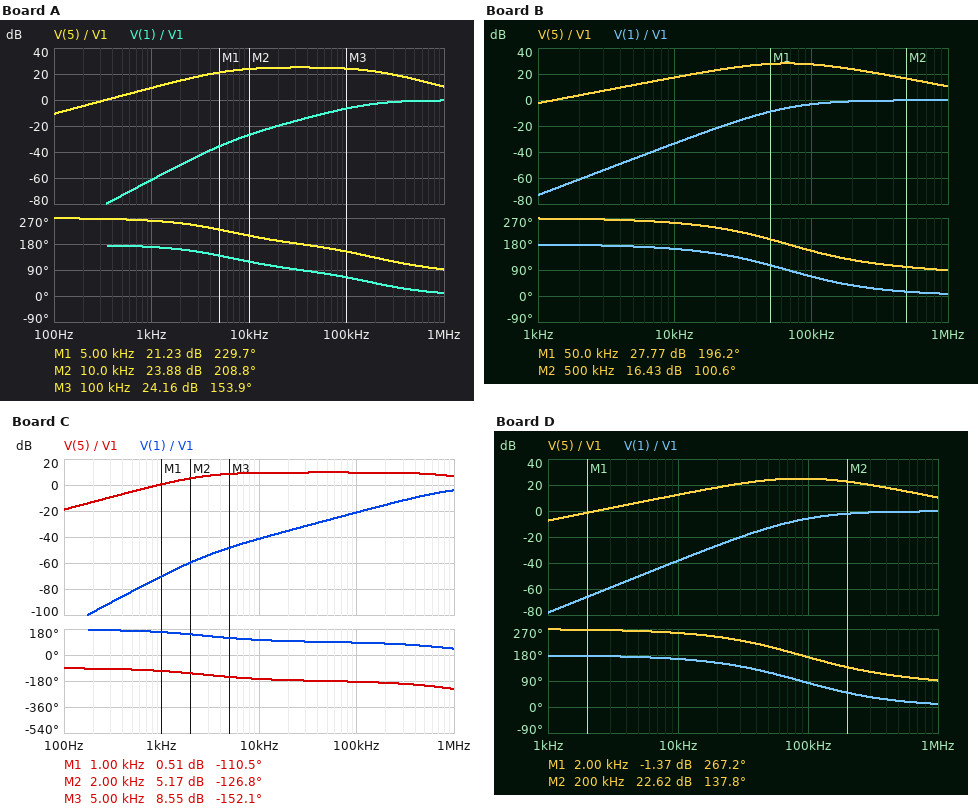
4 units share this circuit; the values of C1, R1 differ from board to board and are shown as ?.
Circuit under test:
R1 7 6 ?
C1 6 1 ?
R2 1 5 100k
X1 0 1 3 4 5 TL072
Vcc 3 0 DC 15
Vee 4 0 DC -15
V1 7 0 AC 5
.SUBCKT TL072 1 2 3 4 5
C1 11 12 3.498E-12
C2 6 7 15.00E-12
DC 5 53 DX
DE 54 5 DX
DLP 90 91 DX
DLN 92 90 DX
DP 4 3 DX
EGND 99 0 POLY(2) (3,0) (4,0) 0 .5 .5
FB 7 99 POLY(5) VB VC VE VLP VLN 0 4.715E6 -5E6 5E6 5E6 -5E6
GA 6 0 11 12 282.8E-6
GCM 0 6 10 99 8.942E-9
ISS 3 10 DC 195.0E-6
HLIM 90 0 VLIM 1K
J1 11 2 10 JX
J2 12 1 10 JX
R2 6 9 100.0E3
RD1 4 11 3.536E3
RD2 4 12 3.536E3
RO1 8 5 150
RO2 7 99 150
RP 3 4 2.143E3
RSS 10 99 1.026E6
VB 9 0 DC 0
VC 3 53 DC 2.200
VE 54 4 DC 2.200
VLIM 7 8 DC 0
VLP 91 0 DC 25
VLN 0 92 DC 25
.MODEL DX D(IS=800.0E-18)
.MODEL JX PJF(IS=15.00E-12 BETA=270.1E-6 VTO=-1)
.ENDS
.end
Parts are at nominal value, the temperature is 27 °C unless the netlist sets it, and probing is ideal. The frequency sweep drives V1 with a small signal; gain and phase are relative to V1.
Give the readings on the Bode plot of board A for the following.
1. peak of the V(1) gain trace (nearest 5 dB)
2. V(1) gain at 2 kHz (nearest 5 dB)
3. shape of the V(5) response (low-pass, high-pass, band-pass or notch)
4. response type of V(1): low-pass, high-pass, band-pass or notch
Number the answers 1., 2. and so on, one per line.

1. 0 dB
2. -50 dB
3. band-pass
4. high-pass
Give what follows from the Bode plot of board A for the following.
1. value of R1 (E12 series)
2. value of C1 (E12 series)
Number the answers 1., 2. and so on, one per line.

1. 5.6 kΩ
2. 4.7 nF
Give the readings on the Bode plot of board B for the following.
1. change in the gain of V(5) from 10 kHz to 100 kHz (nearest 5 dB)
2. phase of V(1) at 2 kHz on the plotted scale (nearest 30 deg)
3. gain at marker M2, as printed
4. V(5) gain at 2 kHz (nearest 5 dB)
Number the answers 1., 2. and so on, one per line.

1. 10 dB
2. 180 deg
3. 16.43 dB
4. 5 dB
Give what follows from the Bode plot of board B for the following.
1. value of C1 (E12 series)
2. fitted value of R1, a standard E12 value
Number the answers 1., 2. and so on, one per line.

1. 1.2 nF
2. 3.9 kΩ
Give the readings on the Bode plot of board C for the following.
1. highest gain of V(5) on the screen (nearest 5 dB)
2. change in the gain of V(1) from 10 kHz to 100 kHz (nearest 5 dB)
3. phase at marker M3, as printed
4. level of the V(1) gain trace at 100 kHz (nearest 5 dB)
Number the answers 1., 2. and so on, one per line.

1. 10 dB
2. 20 dB
3. -152.1 deg
4. -20 dB
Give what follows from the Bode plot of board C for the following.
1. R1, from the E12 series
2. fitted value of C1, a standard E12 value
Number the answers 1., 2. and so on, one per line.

1. 33 kΩ
2. 1.8 nF
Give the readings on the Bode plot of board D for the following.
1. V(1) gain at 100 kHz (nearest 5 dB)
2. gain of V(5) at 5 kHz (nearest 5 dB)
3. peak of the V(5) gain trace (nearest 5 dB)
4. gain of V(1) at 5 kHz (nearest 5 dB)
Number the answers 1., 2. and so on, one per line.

1. -5 dB
2. 5 dB
3. 25 dB
4. -50 dB
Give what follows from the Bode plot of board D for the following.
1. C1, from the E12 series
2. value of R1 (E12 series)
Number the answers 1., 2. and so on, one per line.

1. 680 pF
2. 5.6 kΩ
